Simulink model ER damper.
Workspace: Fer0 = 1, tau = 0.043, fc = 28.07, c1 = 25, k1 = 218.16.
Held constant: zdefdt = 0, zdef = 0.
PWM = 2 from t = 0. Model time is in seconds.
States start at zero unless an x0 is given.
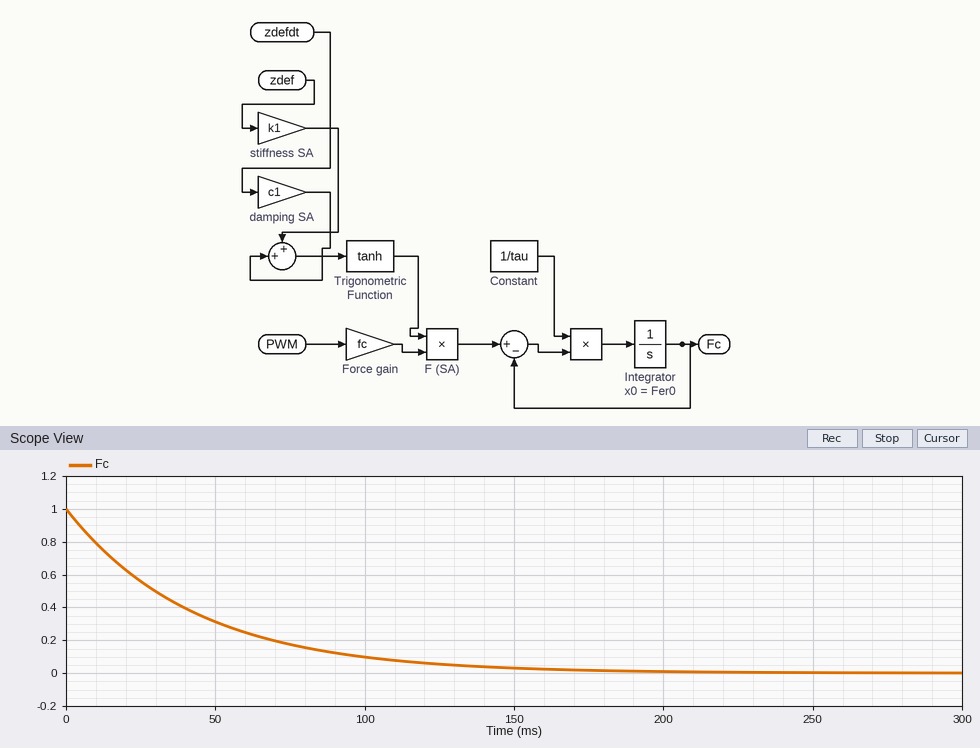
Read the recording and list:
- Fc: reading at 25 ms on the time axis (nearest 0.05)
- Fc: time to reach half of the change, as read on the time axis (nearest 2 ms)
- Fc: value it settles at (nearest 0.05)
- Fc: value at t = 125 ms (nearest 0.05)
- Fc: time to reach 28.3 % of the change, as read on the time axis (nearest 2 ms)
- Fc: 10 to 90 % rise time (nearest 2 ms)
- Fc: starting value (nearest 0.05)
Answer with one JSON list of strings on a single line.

["0.55", "30 ms", "0.00", "0.05", "14 ms", "94 ms", "1.00"]
